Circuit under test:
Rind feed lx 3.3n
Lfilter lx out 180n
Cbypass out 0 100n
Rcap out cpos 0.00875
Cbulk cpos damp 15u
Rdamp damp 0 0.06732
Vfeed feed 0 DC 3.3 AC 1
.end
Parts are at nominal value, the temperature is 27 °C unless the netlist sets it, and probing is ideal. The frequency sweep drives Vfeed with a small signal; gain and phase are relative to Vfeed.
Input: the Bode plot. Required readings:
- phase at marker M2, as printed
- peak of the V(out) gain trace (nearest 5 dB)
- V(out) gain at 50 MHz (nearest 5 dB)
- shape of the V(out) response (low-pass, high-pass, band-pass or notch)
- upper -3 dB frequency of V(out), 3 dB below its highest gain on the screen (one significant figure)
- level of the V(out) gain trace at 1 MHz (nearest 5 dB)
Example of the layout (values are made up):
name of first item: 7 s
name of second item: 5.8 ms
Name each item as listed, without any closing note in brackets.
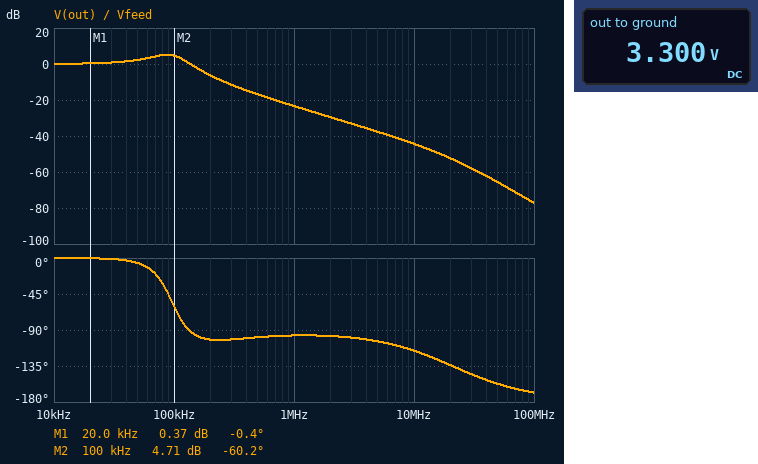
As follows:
phase at marker M2, as printed: -60.2 deg
peak of the V(out) gain trace: 5 dB
V(out) gain at 50 MHz: -65 dB
shape of the V(out) response: low-pass
upper -3 dB frequency of V(out), 3 dB below its highest gain on the screen: 100 kHz
level of the V(out) gain trace at 1 MHz: -25 dB
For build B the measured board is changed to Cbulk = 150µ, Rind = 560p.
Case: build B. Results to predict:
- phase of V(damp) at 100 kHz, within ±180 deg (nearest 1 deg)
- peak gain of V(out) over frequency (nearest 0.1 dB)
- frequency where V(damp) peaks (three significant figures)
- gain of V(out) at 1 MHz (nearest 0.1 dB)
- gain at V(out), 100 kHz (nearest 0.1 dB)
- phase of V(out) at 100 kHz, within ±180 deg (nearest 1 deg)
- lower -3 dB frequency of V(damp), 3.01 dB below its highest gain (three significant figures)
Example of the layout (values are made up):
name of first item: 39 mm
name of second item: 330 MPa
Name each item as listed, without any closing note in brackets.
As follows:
phase of V(damp) at 100 kHz, within ±180 deg: -54 deg
peak gain of V(out) over frequency: 1.1 dB
frequency where V(damp) peaks: 30.7 kHz
gain of V(out) at 1 MHz: -23.4 dB
gain at V(out), 100 kHz: -4.4 dB
phase of V(out) at 100 kHz, within ±180 deg: -62 deg
lower -3 dB frequency of V(damp), 3.01 dB below its highest gain: 11.9 kHz
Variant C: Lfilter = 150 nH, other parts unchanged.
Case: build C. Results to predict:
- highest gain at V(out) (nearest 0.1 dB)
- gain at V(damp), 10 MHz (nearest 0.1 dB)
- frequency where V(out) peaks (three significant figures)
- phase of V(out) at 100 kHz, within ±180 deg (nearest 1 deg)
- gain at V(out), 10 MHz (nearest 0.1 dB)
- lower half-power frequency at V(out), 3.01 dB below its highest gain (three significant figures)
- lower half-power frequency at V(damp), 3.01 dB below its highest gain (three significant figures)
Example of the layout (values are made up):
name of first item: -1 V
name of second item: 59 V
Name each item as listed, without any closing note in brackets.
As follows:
highest gain at V(out): 4.7 dB
gain at V(damp), 10 MHz: -43.8 dB
frequency where V(out) peaks: 95.5 kHz
phase of V(out) at 100 kHz, within ±180 deg: -46 deg
gain at V(out), 10 MHz: -42.8 dB
lower half-power frequency at V(out), 3.01 dB below its highest gain: 47.2 kHz
lower half-power frequency at V(damp), 3.01 dB below its highest gain: 73.3 kHz
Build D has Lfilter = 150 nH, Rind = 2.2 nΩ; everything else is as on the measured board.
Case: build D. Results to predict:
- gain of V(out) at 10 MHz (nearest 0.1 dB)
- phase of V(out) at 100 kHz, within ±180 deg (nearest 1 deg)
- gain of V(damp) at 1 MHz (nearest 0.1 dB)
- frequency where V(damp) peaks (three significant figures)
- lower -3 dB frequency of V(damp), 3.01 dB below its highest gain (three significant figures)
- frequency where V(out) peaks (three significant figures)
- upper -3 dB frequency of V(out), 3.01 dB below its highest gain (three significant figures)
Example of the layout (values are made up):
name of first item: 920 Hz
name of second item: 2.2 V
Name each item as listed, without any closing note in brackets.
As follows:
gain of V(out) at 10 MHz: -42.8 dB
phase of V(out) at 100 kHz, within ±180 deg: -46 deg
gain of V(damp) at 1 MHz: -22.9 dB
frequency where V(damp) peaks: 106 kHz
lower -3 dB frequency of V(damp), 3.01 dB below its highest gain: 73.3 kHz
frequency where V(out) peaks: 95.5 kHz
upper -3 dB frequency of V(out), 3.01 dB below its highest gain: 135 kHz
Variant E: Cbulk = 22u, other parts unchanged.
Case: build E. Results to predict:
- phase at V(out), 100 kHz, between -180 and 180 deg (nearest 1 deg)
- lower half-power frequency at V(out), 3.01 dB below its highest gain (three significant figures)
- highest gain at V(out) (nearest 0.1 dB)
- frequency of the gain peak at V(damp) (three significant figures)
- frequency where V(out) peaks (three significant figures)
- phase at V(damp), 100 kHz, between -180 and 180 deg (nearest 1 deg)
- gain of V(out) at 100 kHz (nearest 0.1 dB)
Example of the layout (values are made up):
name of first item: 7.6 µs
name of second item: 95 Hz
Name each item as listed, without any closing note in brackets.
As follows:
phase at V(out), 100 kHz, between -180 and 180 deg: -72 deg
lower half-power frequency at V(out), 3.01 dB below its highest gain: 29.6 kHz
highest gain at V(out): 4.2 dB
frequency of the gain peak at V(damp): 79.9 kHz
frequency where V(out) peaks: 70.8 kHz
phase at V(damp), 100 kHz, between -180 and 180 deg: -29 deg
gain of V(out) at 100 kHz: 1.7 dB
